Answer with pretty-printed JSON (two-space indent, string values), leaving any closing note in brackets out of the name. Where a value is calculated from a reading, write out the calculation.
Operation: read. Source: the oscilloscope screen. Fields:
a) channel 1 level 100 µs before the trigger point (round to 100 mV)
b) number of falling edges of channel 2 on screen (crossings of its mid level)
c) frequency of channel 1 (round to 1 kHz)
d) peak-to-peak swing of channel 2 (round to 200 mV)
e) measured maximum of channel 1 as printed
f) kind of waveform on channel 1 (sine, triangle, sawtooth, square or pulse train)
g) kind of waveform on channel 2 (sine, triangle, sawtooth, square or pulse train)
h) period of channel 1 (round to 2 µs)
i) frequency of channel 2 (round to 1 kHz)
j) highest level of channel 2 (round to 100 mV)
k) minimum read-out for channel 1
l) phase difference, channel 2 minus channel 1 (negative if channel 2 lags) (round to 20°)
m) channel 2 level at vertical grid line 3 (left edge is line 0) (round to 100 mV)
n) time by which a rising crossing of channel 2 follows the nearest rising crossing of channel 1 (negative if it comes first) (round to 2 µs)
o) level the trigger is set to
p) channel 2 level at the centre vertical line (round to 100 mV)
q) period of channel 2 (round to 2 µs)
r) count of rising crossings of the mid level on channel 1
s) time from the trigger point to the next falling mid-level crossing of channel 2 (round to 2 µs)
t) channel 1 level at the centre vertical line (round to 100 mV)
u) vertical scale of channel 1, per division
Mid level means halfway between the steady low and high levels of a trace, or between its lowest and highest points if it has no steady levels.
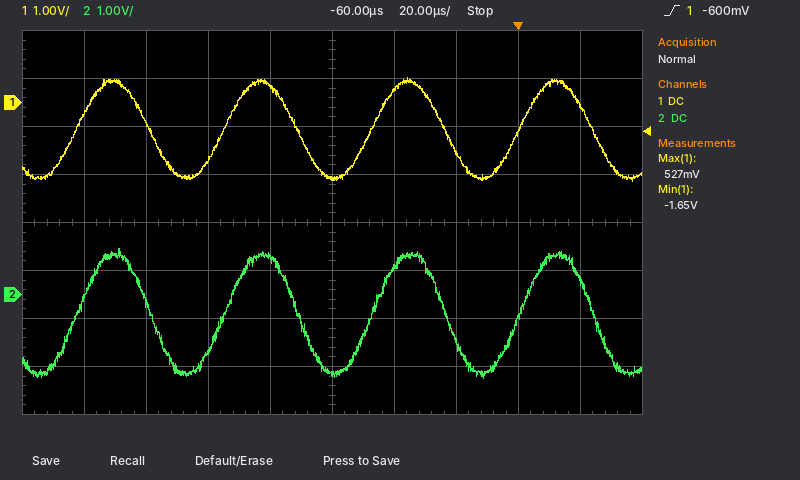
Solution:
{
  "channel 1 level 100 µs before the trigger point": "-1.2 V",
  "number of falling edges of channel 2 on screen": "4",
  "frequency of channel 1": "1 / 48 µs ≈ 21 kHz",
  "peak-to-peak swing of channel 2": "2.8 V",
  "measured maximum of channel 1 as printed": "527 mV",
  "kind of waveform on channel 1": "sine",
  "kind of waveform on channel 2": "sine",
  "period of channel 1": "48 µs",
  "frequency of channel 2": "1 / 48 µs ≈ 21 kHz",
  "highest level of channel 2": "1.0 V",
  "minimum read-out for channel 1": "-1.65 V",
  "phase difference, channel 2 minus channel 1 (negative if channel 2 lags)": "−360° × (0 µs) / 48 µs ≈ 0°",
  "channel 2 level at vertical grid line 3 (left edge is line 0)": "-1.2 V",
  "time by which a rising crossing of channel 2 follows the nearest rising crossing of channel 1 (negative if it comes first)": "0 µs",
  "level the trigger is set to": "-600 mV",
  "channel 2 level at the centre vertical line": "-1.7 V",
  "period of channel 2": "48 µs",
  "count of rising crossings of the mid level on channel 1": "4",
  "time from the trigger point to the next falling mid-level crossing of channel 2": "24 µs",
  "channel 1 level at the centre vertical line": "-1.6 V",
  "vertical scale of channel 1, per division": "1 V"
}
